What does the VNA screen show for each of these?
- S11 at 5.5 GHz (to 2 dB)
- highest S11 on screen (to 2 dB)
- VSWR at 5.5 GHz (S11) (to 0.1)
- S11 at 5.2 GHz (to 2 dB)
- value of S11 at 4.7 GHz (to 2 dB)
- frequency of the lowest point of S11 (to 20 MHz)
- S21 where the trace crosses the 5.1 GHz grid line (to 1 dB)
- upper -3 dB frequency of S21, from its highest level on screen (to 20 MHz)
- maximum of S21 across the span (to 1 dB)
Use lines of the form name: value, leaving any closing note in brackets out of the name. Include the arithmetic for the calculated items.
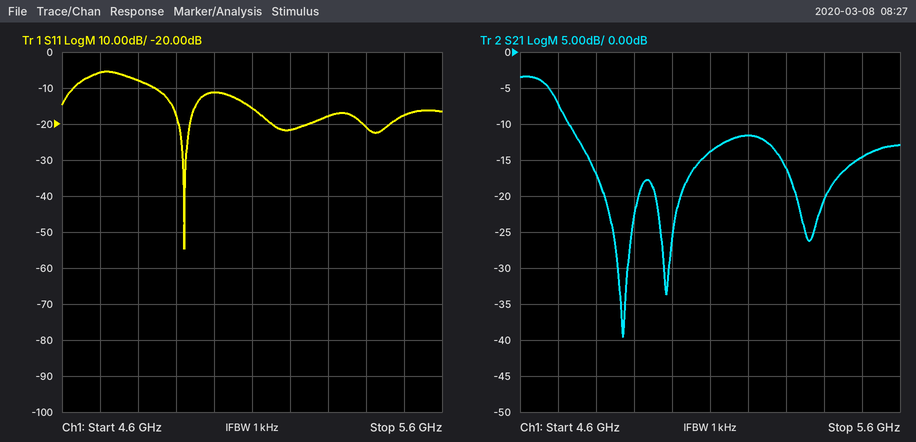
S11 at 5.5 GHz: -18 dB
highest S11 on screen: -6 dB
VSWR at 5.5 GHz (S11): |Γ| = 10^(-18/20) = 0.1259; VSWR = (1 + 0.1259)/(1 − 0.1259) ≈ 1.3
S11 at 5.2 GHz: -22 dB
value of S11 at 4.7 GHz: -6 dB
frequency of the lowest point of S11: 4.92 GHz
S21 where the trace crosses the 5.1 GHz grid line: -14 dB
upper -3 dB frequency of S21, from its highest level on screen: 4.70 GHz
maximum of S21 across the span: -3 dB
